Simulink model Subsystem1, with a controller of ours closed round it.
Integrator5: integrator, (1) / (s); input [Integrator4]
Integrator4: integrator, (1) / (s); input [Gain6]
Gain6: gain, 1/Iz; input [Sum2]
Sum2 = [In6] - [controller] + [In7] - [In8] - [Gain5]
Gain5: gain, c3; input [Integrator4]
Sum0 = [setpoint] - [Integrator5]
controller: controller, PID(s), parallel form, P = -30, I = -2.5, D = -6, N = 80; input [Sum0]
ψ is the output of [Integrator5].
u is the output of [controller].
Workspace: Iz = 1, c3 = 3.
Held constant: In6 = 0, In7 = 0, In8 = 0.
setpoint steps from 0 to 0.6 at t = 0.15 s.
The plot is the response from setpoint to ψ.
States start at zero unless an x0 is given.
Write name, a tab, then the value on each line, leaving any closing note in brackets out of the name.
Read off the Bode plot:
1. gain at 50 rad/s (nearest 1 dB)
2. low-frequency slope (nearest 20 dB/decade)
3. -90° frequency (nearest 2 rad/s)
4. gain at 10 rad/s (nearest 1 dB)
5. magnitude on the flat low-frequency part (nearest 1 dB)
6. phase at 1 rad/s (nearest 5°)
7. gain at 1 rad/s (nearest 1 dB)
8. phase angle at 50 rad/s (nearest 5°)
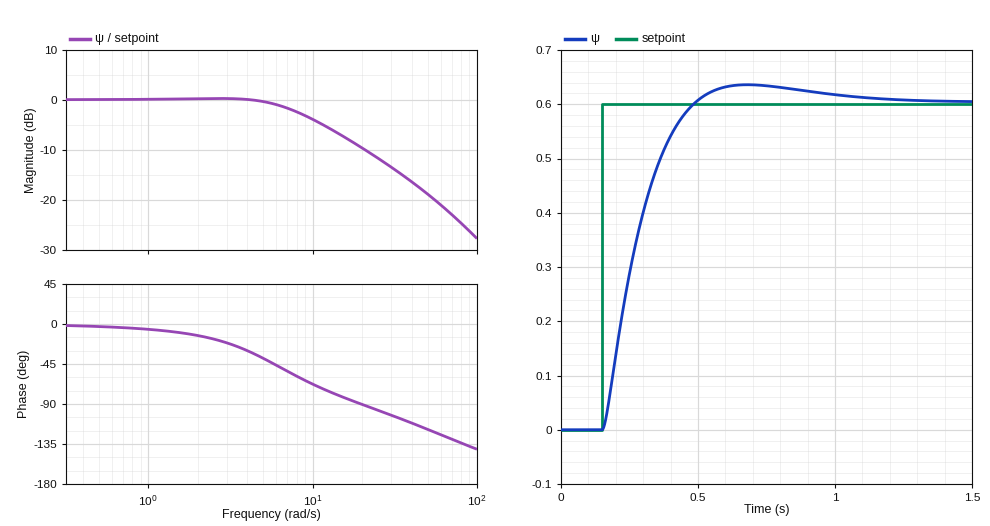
gain at 50 rad/s	-19 dB
low-frequency slope	0 dB/decade
-90° frequency	20 rad/s
gain at 10 rad/s	-4 dB
magnitude on the flat low-frequency part	0 dB
phase at 1 rad/s	-5°
gain at 1 rad/s	0 dB
phase angle at 50 rad/s	-120°
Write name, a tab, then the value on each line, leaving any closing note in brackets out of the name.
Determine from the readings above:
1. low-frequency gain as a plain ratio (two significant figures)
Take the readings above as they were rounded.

low-frequency gain as a plain ratio	1.0
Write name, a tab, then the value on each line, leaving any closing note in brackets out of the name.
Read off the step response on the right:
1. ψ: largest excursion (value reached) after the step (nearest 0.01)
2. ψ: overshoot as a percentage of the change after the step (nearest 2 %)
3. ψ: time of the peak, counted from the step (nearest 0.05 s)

ψ: largest excursion (value reached) after the step	0.64
ψ: overshoot as a percentage of the change after the step	6 %
ψ: time of the peak, counted from the step	0.55 s
